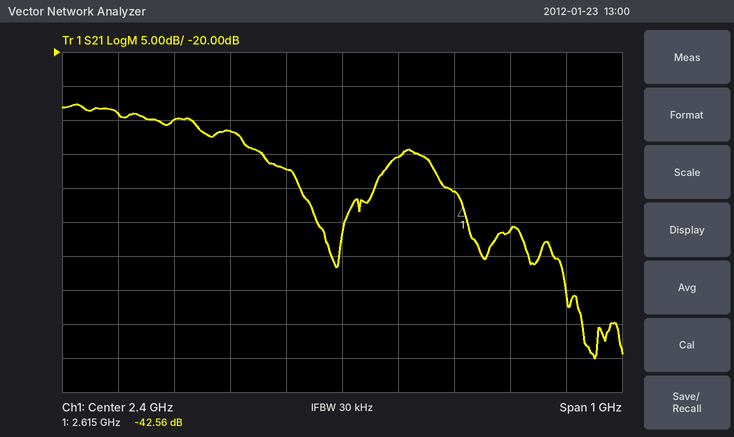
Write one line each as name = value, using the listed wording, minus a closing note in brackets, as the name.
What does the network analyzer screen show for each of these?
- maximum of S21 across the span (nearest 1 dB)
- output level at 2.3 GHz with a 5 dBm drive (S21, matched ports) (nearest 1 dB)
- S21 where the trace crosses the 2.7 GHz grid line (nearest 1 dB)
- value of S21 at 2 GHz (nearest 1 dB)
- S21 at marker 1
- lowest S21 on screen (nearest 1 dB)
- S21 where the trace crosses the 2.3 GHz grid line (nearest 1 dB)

maximum of S21 across the span = -28 dB
output level at 2.3 GHz with a 5 dBm drive (S21, matched ports) = -32 dBm
S21 where the trace crosses the 2.7 GHz grid line = -46 dB
value of S21 at 2 GHz = -29 dB
S21 at marker 1 = -42.56 dB
lowest S21 on screen = -65 dB
S21 where the trace crosses the 2.3 GHz grid line = -37 dB
